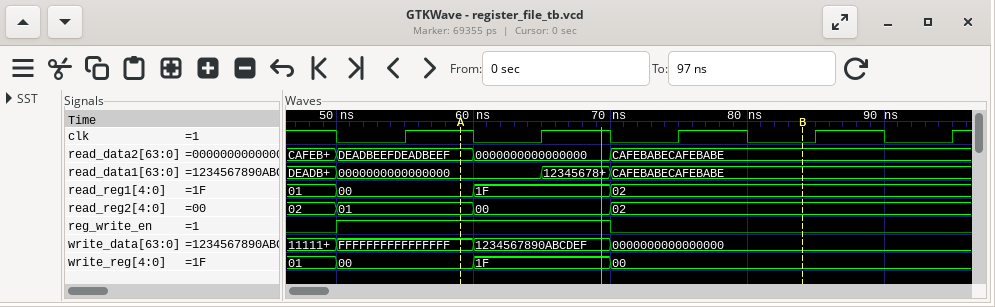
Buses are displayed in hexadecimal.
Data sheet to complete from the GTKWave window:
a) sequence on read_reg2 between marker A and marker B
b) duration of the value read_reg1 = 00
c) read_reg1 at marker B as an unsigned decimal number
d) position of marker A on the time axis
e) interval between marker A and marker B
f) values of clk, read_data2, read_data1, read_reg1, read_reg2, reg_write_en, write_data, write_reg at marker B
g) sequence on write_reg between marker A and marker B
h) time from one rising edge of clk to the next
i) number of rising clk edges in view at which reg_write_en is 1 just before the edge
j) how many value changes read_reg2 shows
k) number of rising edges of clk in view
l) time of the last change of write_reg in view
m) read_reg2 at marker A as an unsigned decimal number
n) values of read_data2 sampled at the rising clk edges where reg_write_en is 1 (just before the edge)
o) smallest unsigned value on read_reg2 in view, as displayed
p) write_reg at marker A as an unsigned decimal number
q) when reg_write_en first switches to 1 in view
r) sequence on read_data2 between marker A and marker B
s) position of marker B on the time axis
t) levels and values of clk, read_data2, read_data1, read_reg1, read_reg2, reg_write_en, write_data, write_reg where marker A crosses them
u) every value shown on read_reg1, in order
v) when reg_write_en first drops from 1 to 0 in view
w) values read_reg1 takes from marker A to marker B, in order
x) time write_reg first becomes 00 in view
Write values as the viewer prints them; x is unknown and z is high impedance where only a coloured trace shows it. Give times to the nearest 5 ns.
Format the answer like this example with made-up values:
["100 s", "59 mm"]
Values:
["01, 00, 02", "10 ns", "2", "60 ns", "25 ns", "clk=0, read_data2=CAFEBABECAFEBABE, read_data1=CAFEBABECAFEBABE, read_reg1=02, read_reg2=02, reg_write_en=0, write_data=0000000000000000, write_reg=00", "00, 1F, 00", "10 ns", "2", "3", "5", "70 ns", "1", "DEADBEEFDEADBEEF, 0000000000000000", "00", "0", "50 ns", "DEADBEEFDEADBEEF, 0000000000000000, CAFEBABECAFEBABE", "85 ns", "clk=1, read_data2=DEADBEEFDEADBEEF, read_data1=0000000000000000, read_reg1=00, read_reg2=01, reg_write_en=1, write_data=FFFFFFFFFFFFFFFF, write_reg=00", "01, 00, 1F, 02", "70 ns", "00, 1F, 02", "50 ns"]
